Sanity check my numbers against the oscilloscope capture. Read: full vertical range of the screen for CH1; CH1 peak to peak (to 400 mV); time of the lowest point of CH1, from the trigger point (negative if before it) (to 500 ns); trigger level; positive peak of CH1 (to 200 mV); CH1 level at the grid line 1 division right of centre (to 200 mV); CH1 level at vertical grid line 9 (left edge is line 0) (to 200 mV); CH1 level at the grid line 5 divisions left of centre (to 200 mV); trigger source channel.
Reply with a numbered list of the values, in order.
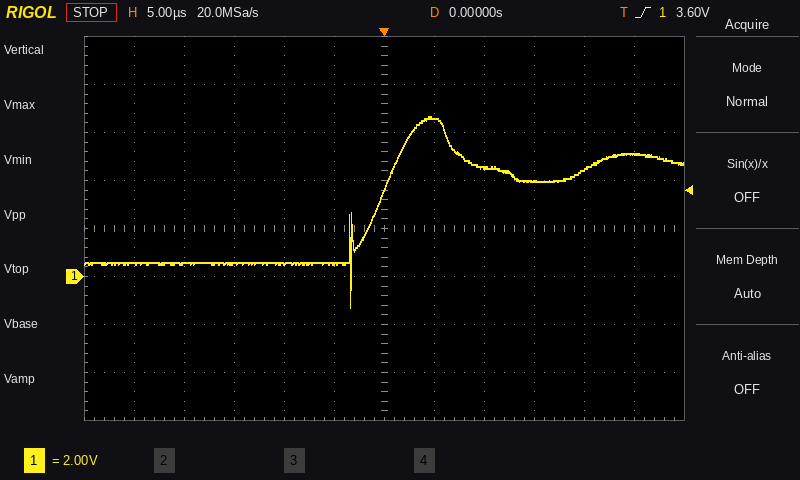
1. 16 V
2. 8.0 V
3. -3.5 µs
4. 3.60 V
5. 6.6 V
6. 6.6 V
7. 4.0 V
8. 600 mV
9. CH1
